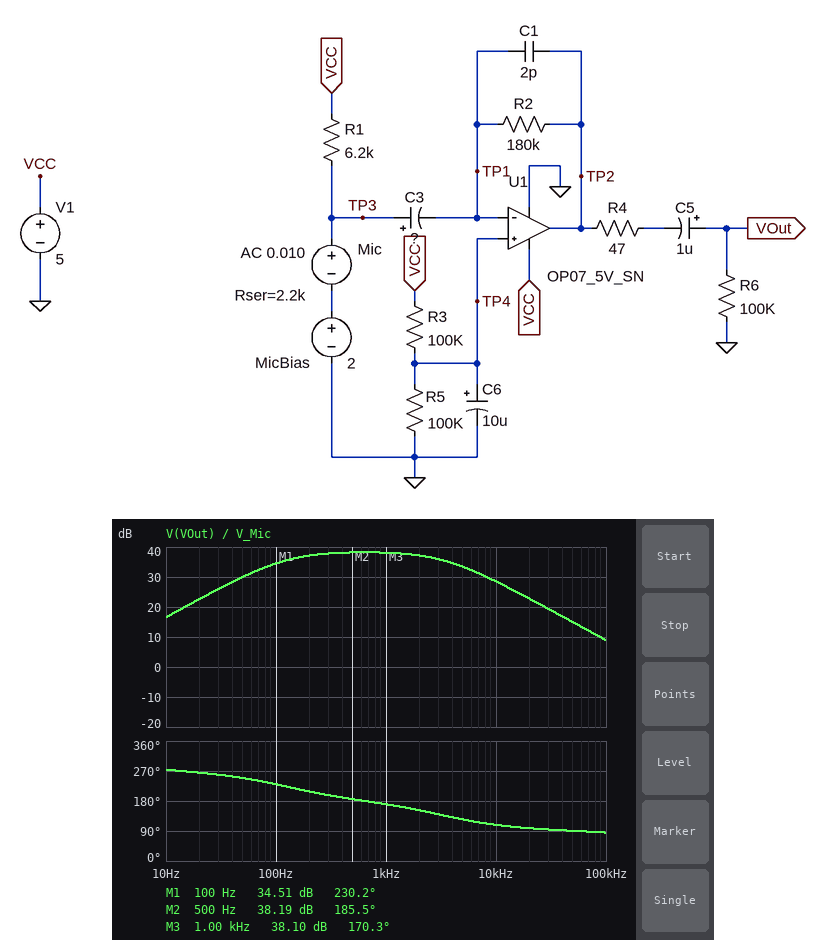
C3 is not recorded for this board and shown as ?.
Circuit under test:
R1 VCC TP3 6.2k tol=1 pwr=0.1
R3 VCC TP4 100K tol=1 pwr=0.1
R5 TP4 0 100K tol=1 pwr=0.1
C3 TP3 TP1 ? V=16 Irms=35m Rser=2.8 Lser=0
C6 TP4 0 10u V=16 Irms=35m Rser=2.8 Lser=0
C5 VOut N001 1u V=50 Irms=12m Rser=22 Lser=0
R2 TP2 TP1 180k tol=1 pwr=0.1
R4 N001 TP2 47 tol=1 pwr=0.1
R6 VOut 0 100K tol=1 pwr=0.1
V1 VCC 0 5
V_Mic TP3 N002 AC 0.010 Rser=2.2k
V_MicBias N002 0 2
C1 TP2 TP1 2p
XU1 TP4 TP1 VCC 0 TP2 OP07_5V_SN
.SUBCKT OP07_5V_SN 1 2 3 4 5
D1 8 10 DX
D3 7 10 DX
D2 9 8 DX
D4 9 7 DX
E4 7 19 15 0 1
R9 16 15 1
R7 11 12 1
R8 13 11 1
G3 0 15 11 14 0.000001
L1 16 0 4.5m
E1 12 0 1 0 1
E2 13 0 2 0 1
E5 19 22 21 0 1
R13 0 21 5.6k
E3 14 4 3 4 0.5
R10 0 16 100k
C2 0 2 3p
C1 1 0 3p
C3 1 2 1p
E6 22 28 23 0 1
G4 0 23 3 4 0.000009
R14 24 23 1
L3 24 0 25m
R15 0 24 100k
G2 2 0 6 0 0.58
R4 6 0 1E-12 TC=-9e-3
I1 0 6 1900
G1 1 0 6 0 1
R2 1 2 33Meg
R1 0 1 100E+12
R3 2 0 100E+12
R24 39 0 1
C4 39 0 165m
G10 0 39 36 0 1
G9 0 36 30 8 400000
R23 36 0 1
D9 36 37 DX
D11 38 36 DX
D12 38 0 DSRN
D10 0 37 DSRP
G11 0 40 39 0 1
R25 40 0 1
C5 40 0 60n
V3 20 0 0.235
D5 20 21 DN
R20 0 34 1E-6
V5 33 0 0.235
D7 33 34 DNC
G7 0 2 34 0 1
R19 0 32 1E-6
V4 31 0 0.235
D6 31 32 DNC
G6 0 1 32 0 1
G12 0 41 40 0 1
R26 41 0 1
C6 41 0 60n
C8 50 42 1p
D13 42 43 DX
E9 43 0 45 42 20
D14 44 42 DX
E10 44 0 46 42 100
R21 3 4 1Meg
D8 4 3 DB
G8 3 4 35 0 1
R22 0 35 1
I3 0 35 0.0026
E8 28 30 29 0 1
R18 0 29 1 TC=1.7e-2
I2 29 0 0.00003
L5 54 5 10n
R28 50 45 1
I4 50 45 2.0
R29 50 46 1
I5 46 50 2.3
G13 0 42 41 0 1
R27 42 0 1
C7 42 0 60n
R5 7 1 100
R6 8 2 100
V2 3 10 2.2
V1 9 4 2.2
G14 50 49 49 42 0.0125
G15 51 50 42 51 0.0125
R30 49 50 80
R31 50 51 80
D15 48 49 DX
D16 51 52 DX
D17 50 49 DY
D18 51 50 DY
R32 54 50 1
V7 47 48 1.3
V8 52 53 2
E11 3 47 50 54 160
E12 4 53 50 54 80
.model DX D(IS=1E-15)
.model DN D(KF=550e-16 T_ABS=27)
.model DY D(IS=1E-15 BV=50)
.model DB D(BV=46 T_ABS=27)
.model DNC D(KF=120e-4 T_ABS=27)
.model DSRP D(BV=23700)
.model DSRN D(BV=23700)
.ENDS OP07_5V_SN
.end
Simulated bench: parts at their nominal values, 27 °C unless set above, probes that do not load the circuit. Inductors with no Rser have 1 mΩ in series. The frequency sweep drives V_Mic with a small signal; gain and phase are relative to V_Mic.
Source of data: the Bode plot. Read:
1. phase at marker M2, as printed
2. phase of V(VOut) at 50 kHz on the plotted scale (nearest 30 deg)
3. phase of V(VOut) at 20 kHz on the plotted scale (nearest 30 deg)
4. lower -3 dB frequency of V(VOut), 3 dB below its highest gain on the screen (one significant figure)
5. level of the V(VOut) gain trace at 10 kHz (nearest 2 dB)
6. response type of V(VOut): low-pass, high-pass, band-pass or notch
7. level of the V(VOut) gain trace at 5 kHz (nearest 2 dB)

185.5 deg
90 deg
90 deg
100 Hz
28 dB
band-pass
34 dB
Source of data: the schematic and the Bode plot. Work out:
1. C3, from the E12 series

820 nF
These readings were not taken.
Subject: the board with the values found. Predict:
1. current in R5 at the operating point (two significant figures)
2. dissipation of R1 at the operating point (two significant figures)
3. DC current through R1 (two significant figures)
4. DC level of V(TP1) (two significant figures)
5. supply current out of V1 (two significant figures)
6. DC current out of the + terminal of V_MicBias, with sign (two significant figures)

25 µA
790 µW
360 µA
2.5 V
3.0 mA
-360 µA
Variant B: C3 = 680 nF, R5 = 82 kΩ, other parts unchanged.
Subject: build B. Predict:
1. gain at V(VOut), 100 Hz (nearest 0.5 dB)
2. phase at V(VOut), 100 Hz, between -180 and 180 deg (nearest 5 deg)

33.5 dB
-125 deg
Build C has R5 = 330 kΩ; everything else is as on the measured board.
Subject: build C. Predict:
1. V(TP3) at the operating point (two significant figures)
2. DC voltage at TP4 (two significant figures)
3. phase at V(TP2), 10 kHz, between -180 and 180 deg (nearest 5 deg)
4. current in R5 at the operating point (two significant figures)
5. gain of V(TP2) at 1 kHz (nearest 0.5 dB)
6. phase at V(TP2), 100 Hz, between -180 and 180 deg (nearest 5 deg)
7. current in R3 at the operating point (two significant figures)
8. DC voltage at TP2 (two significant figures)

2.8 V
3.4 V
0 deg
10 µA
-32.0 dB
10 deg
16 µA
3.9 V
